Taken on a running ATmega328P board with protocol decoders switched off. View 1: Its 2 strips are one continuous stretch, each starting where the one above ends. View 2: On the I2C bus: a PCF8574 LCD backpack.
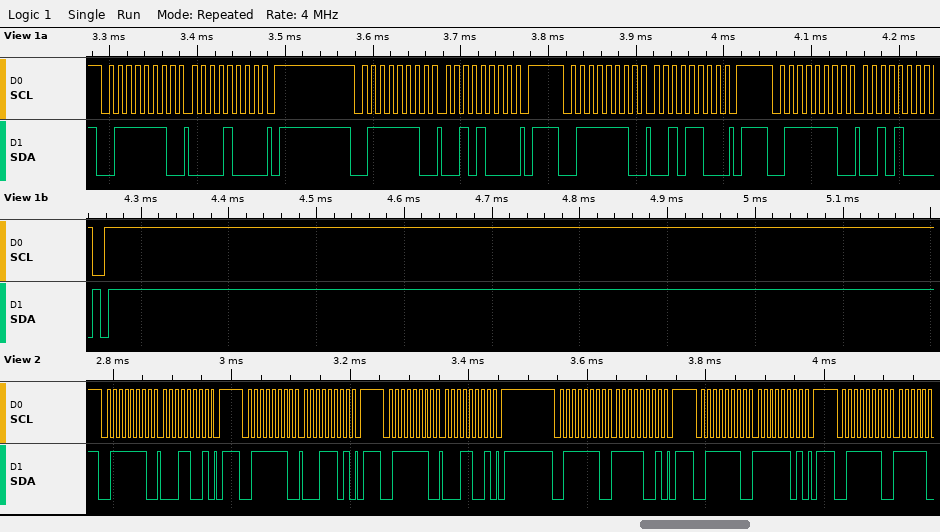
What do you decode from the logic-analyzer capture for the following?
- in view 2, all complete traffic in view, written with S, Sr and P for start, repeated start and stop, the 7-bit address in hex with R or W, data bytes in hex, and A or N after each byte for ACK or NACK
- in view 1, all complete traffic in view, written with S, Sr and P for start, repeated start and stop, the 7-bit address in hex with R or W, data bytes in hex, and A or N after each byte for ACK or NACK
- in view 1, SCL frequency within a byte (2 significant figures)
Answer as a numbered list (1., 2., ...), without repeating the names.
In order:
1. S 3FW A 19 A P S 3FW A 1D A P S 3FW A 19 A P S 3FW A F9 A P S 3FW A FD A P S 3FW A
2. S 3FW A 08 A P S 3FW A 28 A P S 3FW A 2C A P S 3FW A 28 A P
3. 100 kHz
